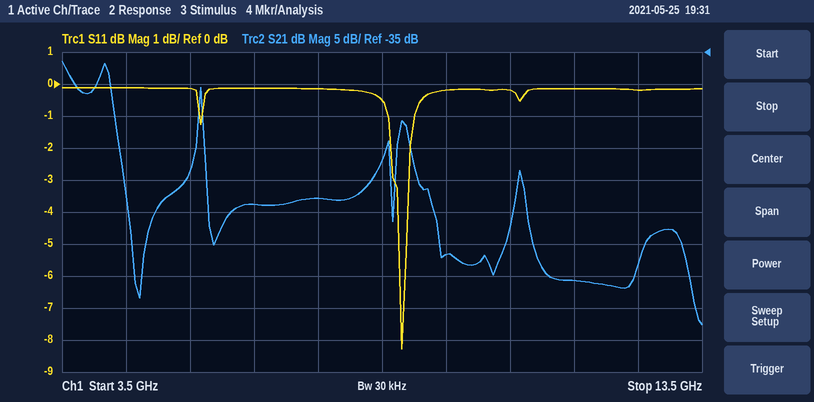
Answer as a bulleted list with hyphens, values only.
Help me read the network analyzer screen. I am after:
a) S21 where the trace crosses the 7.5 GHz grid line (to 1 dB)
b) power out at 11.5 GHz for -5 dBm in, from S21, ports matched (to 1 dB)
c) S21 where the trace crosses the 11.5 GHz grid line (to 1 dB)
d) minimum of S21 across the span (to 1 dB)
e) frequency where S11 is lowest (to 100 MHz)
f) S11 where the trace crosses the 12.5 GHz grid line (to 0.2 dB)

- -58 dB
- -76 dBm
- -71 dB
- -78 dB
- 8.8 GHz
- -0.2 dB
